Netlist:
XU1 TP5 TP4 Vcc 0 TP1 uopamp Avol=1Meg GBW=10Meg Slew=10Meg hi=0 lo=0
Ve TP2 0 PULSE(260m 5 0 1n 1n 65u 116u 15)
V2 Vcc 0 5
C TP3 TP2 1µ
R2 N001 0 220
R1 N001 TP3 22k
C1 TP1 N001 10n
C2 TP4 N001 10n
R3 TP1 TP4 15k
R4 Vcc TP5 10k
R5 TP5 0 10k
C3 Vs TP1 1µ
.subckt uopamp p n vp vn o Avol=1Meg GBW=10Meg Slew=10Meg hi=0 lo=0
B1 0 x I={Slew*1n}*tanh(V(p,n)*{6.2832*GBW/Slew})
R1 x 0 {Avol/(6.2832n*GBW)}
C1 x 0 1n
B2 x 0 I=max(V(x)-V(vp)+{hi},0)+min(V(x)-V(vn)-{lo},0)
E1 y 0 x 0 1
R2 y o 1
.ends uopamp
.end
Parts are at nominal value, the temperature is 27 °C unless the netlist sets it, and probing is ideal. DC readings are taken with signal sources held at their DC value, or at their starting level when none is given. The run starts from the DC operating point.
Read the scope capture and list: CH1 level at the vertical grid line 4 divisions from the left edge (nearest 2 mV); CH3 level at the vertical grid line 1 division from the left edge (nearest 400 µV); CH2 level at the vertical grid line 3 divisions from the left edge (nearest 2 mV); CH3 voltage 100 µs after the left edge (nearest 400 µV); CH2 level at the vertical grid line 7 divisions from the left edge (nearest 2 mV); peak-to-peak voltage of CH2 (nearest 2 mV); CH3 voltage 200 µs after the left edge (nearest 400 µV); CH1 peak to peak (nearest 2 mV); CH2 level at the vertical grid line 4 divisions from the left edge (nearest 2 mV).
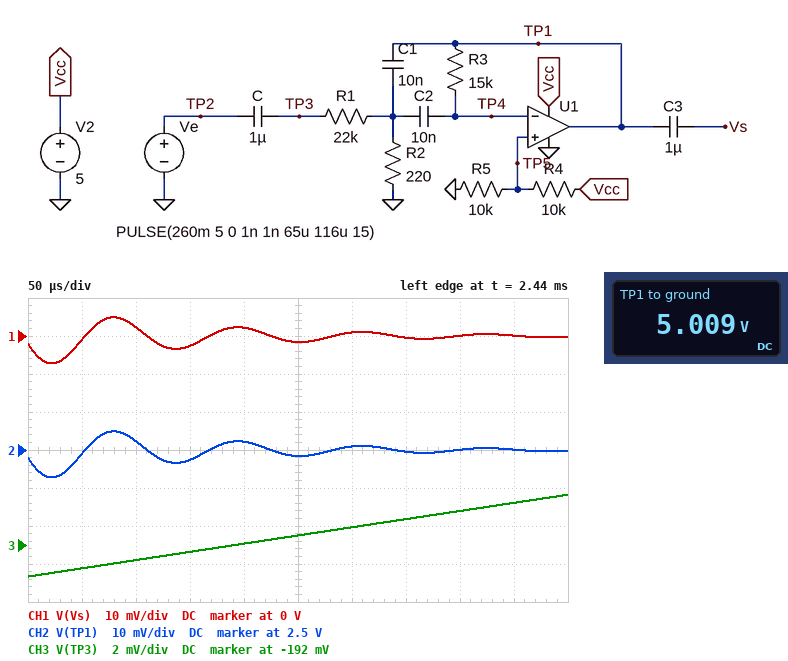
2 mV
-193.2 mV
2.498 V
-192.8 mV
2.500 V
12 mV
-192.0 mV
12 mV
2.502 V
